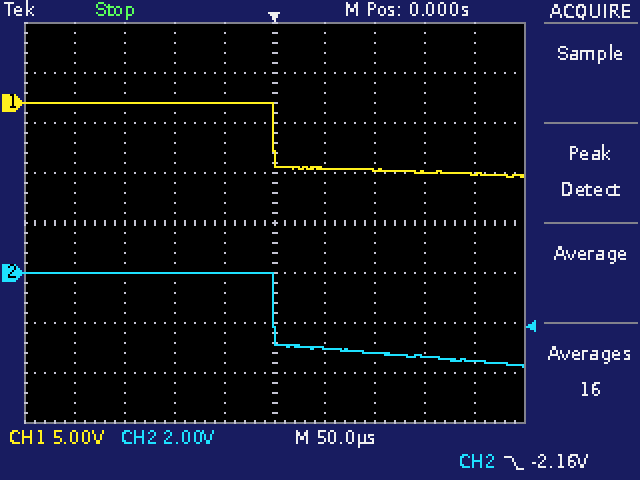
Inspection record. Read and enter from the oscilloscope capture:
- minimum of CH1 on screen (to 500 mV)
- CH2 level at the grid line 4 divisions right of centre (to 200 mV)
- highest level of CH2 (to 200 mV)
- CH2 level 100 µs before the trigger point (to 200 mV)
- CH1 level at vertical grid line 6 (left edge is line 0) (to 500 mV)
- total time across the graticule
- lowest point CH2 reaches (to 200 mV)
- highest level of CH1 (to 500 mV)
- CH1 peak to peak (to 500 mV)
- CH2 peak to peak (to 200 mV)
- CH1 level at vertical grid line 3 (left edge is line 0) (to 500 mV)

-7.5 V
-3.6 V
0.0 V
0.0 V
-6.5 V
500 µs
-3.8 V
0.0 V
7.5 V
3.8 V
0.0 V
